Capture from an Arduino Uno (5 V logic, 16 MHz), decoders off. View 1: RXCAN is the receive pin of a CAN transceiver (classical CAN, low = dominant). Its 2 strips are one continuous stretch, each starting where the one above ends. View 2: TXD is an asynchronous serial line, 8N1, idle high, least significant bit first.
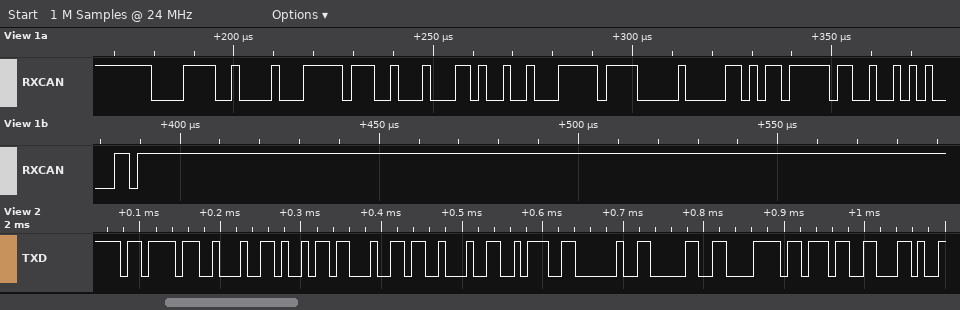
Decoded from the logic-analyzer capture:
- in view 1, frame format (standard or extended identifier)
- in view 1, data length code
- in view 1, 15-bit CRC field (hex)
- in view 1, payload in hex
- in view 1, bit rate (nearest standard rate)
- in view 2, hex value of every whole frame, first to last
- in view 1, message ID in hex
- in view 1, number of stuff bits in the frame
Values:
standard
8
0x12A1
FF 22 34 91 FF 00 2B 7F
500 kbit/s
7B 22 69 64 22 3A 20 30 78 37 2C
0x0F2
5
